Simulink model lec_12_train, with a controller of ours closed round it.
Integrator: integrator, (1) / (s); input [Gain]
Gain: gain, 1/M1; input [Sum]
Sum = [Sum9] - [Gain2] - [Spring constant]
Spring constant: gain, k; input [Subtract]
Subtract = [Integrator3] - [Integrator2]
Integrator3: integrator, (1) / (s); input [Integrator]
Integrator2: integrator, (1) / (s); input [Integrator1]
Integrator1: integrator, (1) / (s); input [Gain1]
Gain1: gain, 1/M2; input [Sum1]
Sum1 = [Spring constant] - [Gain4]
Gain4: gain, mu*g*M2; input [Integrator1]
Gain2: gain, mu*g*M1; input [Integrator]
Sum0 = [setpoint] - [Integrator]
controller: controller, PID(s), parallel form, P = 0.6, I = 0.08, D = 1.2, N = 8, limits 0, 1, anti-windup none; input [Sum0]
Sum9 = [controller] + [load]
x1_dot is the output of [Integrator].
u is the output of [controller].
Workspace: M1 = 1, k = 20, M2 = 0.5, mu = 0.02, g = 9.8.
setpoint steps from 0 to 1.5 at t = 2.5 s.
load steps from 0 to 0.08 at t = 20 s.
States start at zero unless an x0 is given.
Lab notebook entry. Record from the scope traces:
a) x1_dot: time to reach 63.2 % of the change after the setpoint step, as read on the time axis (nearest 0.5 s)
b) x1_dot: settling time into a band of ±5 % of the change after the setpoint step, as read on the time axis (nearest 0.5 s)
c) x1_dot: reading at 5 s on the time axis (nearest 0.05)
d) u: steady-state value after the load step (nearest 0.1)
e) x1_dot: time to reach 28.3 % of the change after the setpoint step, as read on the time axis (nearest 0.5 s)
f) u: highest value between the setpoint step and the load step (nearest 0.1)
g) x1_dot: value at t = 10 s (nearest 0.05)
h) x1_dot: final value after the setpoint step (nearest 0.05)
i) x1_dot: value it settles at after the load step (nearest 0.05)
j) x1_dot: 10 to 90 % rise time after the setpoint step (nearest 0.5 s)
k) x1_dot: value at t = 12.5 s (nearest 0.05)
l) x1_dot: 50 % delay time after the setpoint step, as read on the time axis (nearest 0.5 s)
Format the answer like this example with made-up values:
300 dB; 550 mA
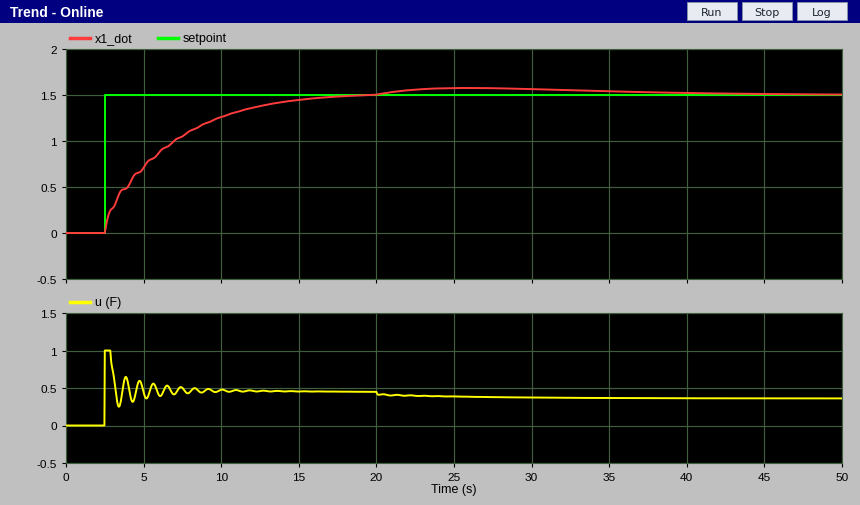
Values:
6.5 s; 14.0 s; 0.70; 0.4; 3.5 s; 1.0; 1.25; 1.50; 1.50; 9.0 s; 1.40; 5.0 s
